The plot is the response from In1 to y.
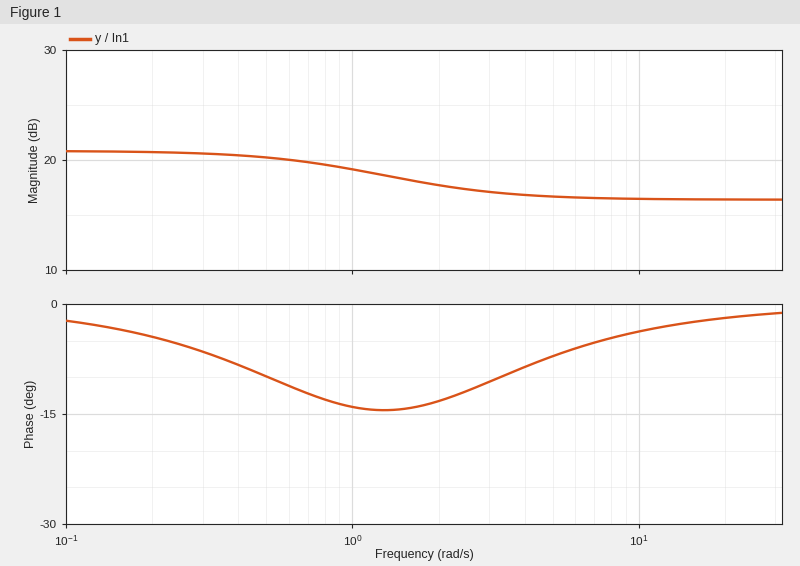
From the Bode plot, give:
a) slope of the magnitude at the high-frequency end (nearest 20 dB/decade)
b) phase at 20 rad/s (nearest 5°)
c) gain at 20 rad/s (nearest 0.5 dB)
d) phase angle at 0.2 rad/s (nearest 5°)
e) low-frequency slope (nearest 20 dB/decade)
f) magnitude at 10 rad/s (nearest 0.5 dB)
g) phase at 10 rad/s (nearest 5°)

0 dB/decade
0°
16.5 dB
-5°
0 dB/decade
16.5 dB
-5°
